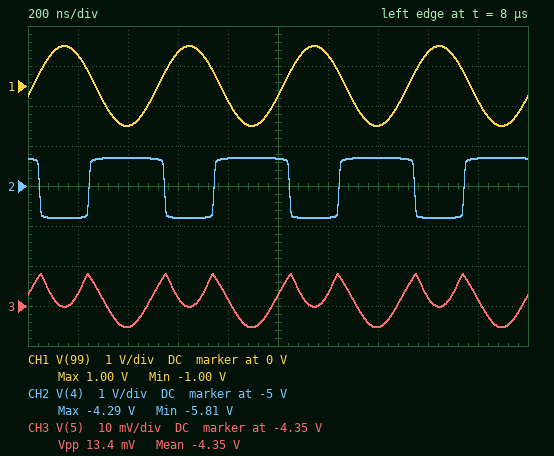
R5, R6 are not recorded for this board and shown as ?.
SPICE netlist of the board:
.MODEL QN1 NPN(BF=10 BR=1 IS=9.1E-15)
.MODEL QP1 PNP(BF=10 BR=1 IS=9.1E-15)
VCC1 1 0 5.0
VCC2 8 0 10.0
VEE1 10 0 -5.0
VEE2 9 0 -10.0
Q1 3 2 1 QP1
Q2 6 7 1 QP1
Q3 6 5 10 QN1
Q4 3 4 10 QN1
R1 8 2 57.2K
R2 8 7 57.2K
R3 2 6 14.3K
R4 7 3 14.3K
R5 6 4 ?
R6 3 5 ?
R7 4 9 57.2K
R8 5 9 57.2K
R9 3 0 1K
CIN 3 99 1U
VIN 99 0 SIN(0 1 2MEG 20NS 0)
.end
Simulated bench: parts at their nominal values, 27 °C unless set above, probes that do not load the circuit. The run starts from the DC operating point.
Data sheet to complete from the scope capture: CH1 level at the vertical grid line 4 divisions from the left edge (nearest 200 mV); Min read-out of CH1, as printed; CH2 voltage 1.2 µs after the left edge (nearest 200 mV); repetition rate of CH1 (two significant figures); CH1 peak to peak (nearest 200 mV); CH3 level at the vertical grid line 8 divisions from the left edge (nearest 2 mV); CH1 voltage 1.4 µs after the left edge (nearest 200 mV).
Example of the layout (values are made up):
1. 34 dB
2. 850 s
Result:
1. -400 mV
2. -1.00 V
3. -5.8 V
4. 2.0 MHz
5. 2.0 V
6. -4.348 V
7. -1.0 V
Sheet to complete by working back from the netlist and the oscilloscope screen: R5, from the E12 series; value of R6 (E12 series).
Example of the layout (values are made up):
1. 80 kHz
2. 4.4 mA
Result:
1. 12 kΩ
2. 33 kΩ
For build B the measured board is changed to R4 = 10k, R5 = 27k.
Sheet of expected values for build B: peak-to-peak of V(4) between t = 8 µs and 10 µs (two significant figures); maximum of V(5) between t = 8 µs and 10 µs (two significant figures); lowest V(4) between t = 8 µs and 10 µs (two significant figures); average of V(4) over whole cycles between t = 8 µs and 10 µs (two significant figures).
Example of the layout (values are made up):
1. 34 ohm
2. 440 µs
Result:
1. 2.2 V
2. -4.3 V
3. -6.6 V
4. -5.3 V
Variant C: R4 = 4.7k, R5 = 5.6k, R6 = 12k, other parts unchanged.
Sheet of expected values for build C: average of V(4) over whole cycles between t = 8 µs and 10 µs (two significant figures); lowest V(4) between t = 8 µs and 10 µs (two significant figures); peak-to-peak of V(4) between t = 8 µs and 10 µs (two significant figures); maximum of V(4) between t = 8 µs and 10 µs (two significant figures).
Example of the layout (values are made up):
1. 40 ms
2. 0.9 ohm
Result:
1. -4.8 V
2. -5.4 V
3. 1.1 V
4. -4.3 V
